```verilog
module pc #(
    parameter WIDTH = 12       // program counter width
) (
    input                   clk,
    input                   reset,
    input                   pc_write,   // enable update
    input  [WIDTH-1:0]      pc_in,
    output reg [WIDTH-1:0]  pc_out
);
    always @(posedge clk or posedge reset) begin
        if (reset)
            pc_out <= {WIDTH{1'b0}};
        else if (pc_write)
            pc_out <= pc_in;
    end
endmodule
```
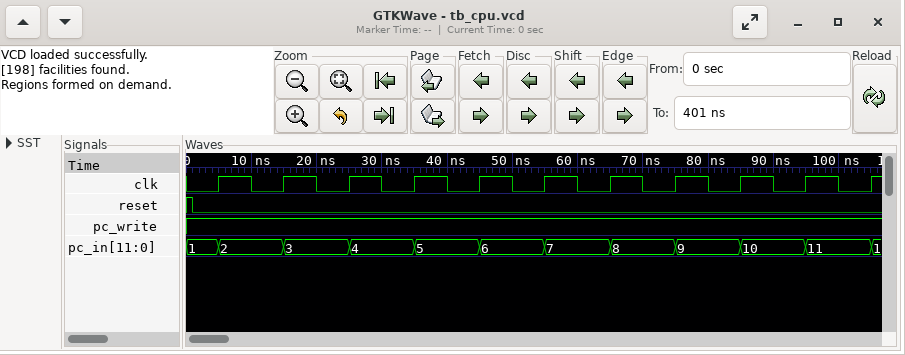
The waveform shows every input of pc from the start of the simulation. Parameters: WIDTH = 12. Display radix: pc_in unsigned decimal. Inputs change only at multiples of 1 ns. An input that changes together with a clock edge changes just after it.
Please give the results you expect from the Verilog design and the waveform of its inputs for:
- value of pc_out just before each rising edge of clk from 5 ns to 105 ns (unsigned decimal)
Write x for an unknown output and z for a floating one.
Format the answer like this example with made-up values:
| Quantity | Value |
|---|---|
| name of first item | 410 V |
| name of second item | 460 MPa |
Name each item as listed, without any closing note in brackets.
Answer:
| Quantity | Value |
|---|---|
| value of pc_out just before each rising edge of clk from 5 ns to 105 ns | 0, 1, 2, 3, 4, 5, 6, 7, 8, 9, 10 |
